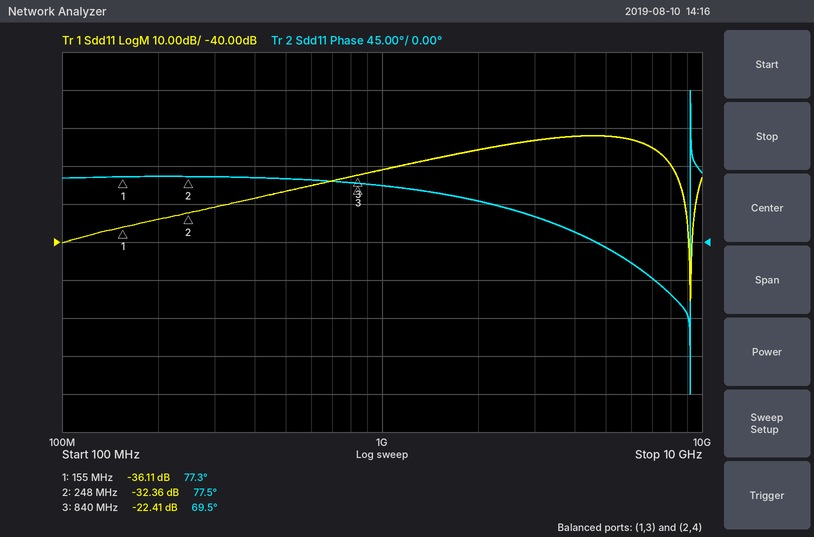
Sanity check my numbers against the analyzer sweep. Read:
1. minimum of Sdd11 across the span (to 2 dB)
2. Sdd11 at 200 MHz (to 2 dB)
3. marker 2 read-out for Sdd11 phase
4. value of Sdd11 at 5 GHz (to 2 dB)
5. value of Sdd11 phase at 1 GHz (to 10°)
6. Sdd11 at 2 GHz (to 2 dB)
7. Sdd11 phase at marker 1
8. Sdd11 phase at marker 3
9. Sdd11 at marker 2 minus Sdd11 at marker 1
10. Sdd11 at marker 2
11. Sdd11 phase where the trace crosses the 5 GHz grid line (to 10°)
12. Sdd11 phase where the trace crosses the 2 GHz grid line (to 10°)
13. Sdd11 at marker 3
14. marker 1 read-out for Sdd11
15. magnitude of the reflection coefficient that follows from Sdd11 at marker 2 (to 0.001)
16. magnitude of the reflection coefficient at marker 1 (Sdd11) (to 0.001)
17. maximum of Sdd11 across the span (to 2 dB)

-56 dB
-34 dB
77.5°
-12 dB
70°
-16 dB
77.3°
69.5°
3.75 dB
-32.36 dB
-10°
50°
-22.41 dB
-36.11 dB
0.024
0.016
-12 dB
